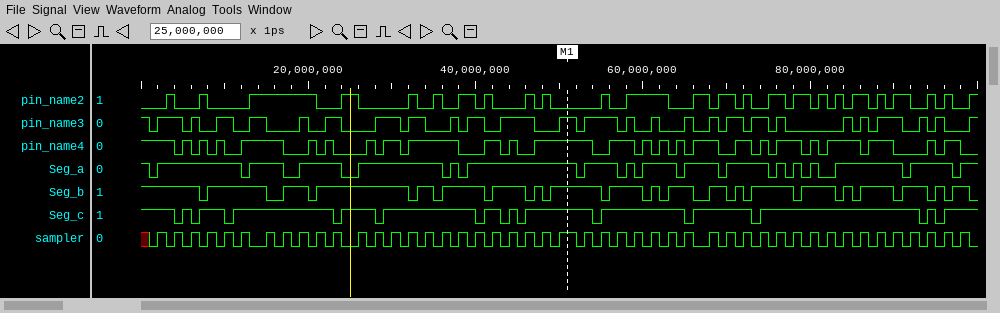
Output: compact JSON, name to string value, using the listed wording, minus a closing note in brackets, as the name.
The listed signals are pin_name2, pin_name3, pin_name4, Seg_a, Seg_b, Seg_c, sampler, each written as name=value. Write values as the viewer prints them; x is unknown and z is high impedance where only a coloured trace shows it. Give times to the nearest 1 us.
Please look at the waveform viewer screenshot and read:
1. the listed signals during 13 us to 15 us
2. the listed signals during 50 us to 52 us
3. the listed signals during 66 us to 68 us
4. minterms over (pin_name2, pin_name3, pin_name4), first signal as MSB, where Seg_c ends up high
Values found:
{"the listed signals during 13 us to 15 us": "pin_name2=1, pin_name3=1, pin_name4=1, Seg_a=1, Seg_b=1, Seg_c=1, sampler=0", "the listed signals during 50 us to 52 us": "pin_name2=0, pin_name3=1, pin_name4=1, Seg_a=1, Seg_b=1, Seg_c=1, sampler=1", "the listed signals during 66 us to 68 us": "pin_name2=1, pin_name3=0, pin_name4=1, Seg_a=1, Seg_b=0, Seg_c=1, sampler=0", "minterms over (pin_name2, pin_name3, pin_name4), first signal as MSB, where Seg_c ends up high": "0, 1, 3, 4, 5, 6, 7"}
